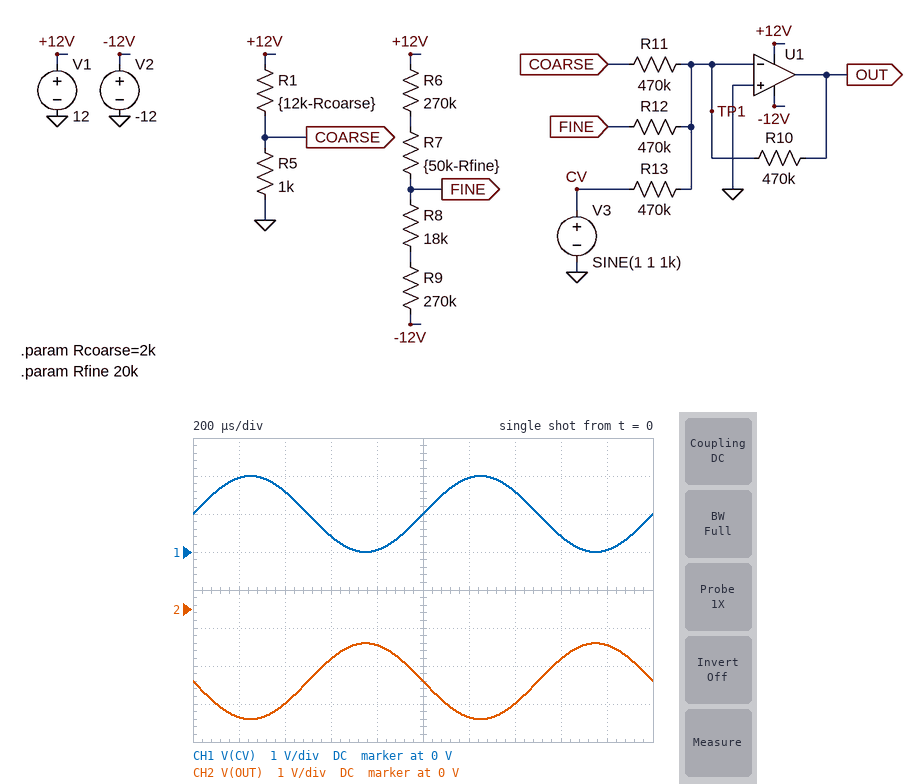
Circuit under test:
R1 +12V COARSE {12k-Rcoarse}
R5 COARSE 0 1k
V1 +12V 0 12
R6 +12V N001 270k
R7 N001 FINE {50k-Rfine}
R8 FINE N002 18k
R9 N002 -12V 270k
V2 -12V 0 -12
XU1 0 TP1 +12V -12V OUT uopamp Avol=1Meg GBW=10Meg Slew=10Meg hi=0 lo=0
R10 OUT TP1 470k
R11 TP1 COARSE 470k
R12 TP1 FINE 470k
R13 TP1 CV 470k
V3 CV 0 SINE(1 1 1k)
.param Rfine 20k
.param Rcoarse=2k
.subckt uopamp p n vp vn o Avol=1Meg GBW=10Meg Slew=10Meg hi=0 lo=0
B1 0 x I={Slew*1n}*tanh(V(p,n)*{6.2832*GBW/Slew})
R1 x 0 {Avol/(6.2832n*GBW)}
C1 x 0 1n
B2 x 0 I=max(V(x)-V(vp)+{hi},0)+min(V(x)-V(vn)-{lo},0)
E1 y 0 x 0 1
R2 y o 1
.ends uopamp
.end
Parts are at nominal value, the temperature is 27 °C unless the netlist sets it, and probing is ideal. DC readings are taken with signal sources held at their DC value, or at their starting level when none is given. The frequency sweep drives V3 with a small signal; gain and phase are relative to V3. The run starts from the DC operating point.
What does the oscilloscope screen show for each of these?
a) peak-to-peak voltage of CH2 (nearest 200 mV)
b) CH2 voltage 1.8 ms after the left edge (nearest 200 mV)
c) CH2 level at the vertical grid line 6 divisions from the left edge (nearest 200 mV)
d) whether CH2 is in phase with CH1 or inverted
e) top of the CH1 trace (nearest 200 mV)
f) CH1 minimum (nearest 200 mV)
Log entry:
2.0 V
-1.0 V
-2.8 V
inverted
2.0 V
0 V
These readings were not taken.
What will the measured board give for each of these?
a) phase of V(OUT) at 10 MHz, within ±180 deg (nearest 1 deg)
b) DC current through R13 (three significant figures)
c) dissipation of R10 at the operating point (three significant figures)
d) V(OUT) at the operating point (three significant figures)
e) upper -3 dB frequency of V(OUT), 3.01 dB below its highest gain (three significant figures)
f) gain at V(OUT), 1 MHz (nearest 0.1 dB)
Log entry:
105 deg
2.13 µA
7.70 µW
-1.90 V
2.66 MHz
-0.6 dB
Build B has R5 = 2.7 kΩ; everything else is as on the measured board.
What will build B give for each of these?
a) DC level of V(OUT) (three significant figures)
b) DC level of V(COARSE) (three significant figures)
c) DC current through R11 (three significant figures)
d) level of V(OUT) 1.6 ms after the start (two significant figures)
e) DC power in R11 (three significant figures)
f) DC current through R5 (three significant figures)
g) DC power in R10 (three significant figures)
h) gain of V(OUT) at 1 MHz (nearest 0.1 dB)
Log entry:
-3.35 V
2.54 V
5.40 µA
-2.8 V
13.7 µW
941 µA
23.9 µW
-0.6 dB
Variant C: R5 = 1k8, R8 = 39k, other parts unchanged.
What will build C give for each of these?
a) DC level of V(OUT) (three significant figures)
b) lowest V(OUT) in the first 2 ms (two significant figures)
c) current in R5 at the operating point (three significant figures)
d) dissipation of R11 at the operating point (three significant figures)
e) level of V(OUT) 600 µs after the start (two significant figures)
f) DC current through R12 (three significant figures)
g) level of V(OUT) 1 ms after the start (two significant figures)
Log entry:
-2.96 V
-4.0 V
1.01 mA
7.08 µW
-2.4 V
285 nA
-3.0 V
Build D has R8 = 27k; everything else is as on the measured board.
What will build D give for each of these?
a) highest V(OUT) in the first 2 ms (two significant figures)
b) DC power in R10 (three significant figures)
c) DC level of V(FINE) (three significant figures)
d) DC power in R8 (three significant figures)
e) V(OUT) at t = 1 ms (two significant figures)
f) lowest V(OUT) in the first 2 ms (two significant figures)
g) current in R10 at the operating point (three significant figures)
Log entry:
-1.0 V
8.88 µW
-45.8 mV
43.7 µW
-2.0 V
-3.0 V
4.35 µA
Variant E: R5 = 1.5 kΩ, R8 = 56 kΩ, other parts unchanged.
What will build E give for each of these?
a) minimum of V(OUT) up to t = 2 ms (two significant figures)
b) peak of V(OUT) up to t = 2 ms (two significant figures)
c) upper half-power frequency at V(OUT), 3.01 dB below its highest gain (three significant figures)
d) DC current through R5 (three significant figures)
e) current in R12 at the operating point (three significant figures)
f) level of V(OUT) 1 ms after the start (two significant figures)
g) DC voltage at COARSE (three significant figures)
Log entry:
-3.9 V
-1.9 V
2.67 MHz
1.04 mA
796 nA
-2.9 V
1.56 V
